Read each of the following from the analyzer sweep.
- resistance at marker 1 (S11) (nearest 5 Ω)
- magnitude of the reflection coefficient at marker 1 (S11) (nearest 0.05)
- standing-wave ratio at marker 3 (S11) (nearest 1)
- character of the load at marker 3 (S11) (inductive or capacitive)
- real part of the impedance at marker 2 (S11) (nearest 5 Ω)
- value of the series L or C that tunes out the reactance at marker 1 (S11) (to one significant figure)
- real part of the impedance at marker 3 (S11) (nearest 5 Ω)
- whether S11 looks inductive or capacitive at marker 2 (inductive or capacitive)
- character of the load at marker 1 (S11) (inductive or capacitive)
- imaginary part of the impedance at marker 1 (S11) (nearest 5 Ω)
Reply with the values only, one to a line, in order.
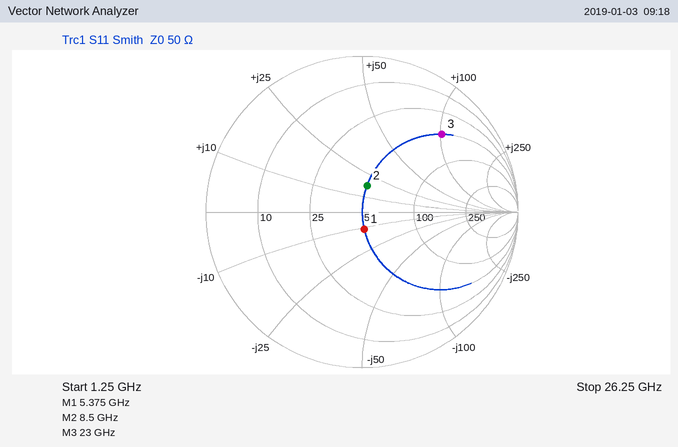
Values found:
50 Ω
0.10
6
inductive
50 Ω
300 pH
50 Ω
inductive
capacitive
-10 Ω
